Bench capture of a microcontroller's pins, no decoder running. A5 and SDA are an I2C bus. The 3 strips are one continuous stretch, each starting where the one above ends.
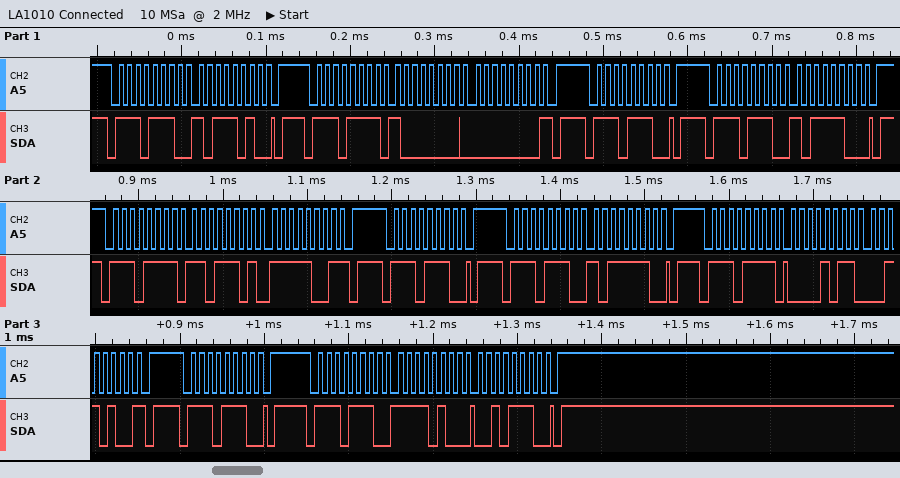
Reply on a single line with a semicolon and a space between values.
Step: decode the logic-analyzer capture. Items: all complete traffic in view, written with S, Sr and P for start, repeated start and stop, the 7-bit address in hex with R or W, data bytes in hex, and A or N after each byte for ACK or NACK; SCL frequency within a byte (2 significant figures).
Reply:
S 77W A BA A P S 77R A 80 A 00 N P S 77W A P S 77W A BC A P S 77R A DD A F9 N P S 77W A P S 77W A BE A P S 77R A 0B A 34 N P S 77W A P S 77W A F4 A 2E A P; 100 kHz
